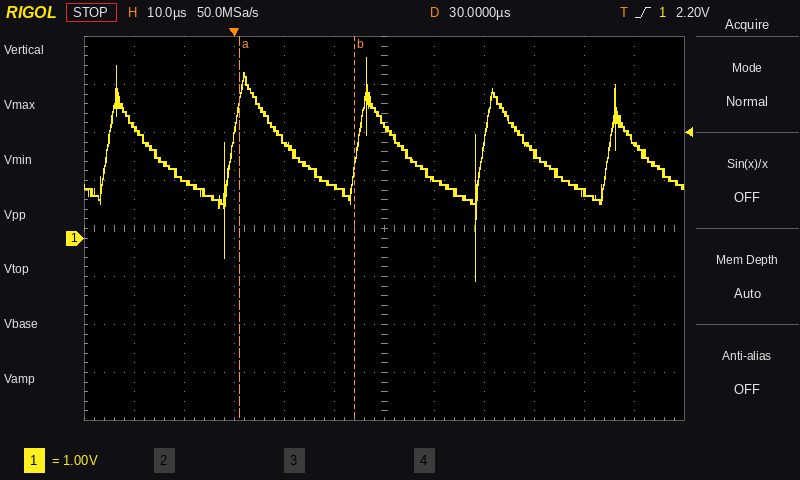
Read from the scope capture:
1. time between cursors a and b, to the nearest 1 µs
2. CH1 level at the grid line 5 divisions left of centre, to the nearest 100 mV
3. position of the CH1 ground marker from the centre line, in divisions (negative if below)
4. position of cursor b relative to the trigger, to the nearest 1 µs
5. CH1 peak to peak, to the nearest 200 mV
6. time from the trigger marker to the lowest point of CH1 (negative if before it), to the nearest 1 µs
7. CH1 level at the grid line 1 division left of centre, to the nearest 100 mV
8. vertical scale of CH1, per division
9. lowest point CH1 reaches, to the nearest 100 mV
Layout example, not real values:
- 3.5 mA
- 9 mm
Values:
- 23 µs
- 2.3 V
- -0.2 div
- +24 µs
- 4.6 V
- +48 µs
- 1.1 V
- 1 V
- -900 mV
